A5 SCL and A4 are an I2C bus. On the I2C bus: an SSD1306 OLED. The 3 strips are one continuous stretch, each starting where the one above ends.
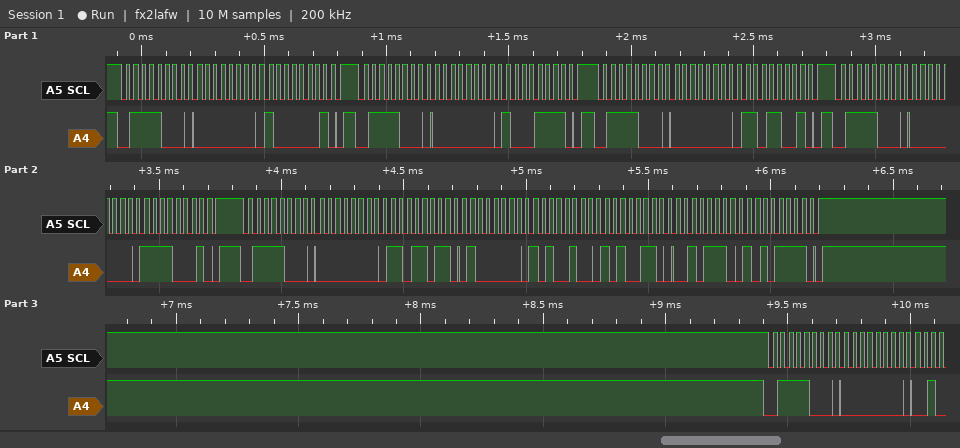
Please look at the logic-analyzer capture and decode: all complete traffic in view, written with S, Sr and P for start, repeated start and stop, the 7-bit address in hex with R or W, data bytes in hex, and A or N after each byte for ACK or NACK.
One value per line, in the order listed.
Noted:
S 3CW A 00 A 81 A P S 3CW A 00 A 8F A P S 3CW A 00 A D9 A P S 3CW A 00 A F1 A P S 3CW A 00 A DB A 40 A A4 A A6 A 2E A AF A P S 3CW A 00 A
